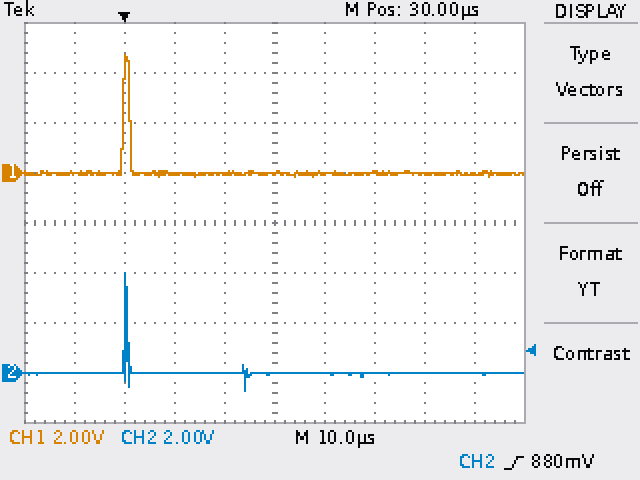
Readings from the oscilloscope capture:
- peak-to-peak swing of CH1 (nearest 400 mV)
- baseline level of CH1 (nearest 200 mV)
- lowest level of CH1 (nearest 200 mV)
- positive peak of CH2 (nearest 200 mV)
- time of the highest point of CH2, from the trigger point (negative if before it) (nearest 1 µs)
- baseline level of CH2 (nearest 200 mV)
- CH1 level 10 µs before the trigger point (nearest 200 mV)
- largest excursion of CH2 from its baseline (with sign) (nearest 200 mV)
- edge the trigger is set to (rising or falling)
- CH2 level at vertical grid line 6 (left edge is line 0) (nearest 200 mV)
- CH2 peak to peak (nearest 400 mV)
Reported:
4.8 V
0.0 V
-200 mV
4.0 V
0 µs
0.0 V
0.0 V
+4.0 V
rising
0.0 V
4.8 V
